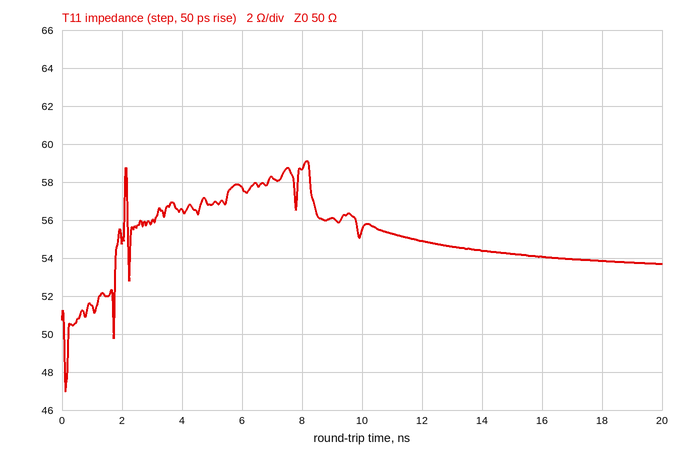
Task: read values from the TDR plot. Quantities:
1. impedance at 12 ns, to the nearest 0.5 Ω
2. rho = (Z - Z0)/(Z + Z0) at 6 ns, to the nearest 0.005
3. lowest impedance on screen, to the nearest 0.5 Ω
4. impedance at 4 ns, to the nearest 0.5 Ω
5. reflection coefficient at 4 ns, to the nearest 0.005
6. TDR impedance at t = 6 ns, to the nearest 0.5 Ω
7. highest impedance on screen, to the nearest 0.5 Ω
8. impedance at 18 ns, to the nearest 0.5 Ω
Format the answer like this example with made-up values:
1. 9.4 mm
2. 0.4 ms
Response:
1. 55.0 Ω
2. +0.070
3. 47.0 Ω
4. 56.5 Ω
5. +0.060
6. 57.5 Ω
7. 59.0 Ω
8. 54.0 Ω
